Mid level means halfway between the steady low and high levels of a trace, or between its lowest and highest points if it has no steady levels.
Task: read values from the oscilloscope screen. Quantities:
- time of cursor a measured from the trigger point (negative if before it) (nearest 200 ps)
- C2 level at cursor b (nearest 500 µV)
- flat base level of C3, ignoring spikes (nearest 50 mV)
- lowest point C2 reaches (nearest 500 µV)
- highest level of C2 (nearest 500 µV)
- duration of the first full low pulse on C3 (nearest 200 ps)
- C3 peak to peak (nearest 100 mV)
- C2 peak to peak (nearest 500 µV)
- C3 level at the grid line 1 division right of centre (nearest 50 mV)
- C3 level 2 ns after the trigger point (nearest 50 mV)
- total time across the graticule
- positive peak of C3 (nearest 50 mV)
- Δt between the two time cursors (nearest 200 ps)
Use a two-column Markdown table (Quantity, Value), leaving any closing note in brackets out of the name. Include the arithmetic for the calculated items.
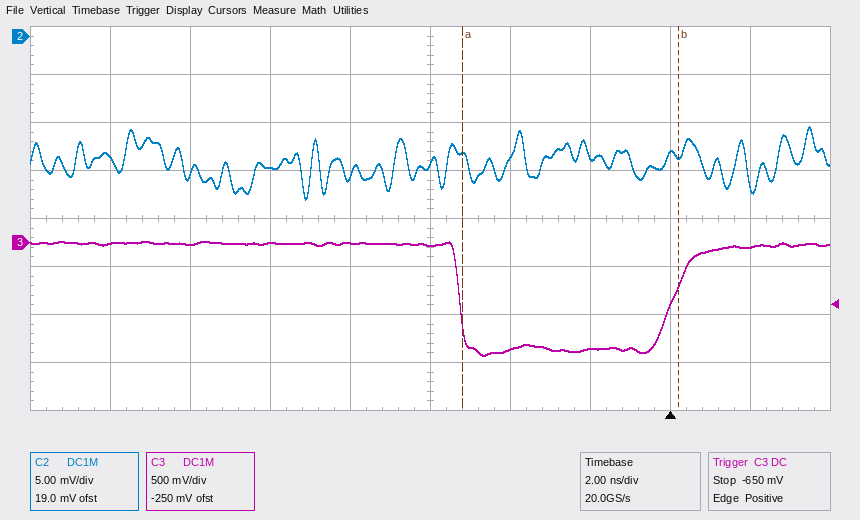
| Quantity | Value |
|---|---|
| time of cursor a measured from the trigger point (negative if before it) | -5.2 ns |
| C2 level at cursor b | -12.5 mV |
| flat base level of C3, ignoring spikes | -1.10 V |
| lowest point C2 reaches | -17.0 mV |
| highest level of C2 | -9.5 mV |
| duration of the first full low pulse on C3 | 5.4 ns |
| C3 peak to peak | 1.20 V |
| C2 peak to peak | -9.5 mV − (-17.0 mV) = 7.5 mV |
| C3 level at the grid line 1 division right of centre | -1.10 V |
| C3 level 2 ns after the trigger point | -50 mV |
| total time across the graticule | 20 ns |
| positive peak of C3 | 0 mV |
| Δt between the two time cursors | 5.4 ns |
